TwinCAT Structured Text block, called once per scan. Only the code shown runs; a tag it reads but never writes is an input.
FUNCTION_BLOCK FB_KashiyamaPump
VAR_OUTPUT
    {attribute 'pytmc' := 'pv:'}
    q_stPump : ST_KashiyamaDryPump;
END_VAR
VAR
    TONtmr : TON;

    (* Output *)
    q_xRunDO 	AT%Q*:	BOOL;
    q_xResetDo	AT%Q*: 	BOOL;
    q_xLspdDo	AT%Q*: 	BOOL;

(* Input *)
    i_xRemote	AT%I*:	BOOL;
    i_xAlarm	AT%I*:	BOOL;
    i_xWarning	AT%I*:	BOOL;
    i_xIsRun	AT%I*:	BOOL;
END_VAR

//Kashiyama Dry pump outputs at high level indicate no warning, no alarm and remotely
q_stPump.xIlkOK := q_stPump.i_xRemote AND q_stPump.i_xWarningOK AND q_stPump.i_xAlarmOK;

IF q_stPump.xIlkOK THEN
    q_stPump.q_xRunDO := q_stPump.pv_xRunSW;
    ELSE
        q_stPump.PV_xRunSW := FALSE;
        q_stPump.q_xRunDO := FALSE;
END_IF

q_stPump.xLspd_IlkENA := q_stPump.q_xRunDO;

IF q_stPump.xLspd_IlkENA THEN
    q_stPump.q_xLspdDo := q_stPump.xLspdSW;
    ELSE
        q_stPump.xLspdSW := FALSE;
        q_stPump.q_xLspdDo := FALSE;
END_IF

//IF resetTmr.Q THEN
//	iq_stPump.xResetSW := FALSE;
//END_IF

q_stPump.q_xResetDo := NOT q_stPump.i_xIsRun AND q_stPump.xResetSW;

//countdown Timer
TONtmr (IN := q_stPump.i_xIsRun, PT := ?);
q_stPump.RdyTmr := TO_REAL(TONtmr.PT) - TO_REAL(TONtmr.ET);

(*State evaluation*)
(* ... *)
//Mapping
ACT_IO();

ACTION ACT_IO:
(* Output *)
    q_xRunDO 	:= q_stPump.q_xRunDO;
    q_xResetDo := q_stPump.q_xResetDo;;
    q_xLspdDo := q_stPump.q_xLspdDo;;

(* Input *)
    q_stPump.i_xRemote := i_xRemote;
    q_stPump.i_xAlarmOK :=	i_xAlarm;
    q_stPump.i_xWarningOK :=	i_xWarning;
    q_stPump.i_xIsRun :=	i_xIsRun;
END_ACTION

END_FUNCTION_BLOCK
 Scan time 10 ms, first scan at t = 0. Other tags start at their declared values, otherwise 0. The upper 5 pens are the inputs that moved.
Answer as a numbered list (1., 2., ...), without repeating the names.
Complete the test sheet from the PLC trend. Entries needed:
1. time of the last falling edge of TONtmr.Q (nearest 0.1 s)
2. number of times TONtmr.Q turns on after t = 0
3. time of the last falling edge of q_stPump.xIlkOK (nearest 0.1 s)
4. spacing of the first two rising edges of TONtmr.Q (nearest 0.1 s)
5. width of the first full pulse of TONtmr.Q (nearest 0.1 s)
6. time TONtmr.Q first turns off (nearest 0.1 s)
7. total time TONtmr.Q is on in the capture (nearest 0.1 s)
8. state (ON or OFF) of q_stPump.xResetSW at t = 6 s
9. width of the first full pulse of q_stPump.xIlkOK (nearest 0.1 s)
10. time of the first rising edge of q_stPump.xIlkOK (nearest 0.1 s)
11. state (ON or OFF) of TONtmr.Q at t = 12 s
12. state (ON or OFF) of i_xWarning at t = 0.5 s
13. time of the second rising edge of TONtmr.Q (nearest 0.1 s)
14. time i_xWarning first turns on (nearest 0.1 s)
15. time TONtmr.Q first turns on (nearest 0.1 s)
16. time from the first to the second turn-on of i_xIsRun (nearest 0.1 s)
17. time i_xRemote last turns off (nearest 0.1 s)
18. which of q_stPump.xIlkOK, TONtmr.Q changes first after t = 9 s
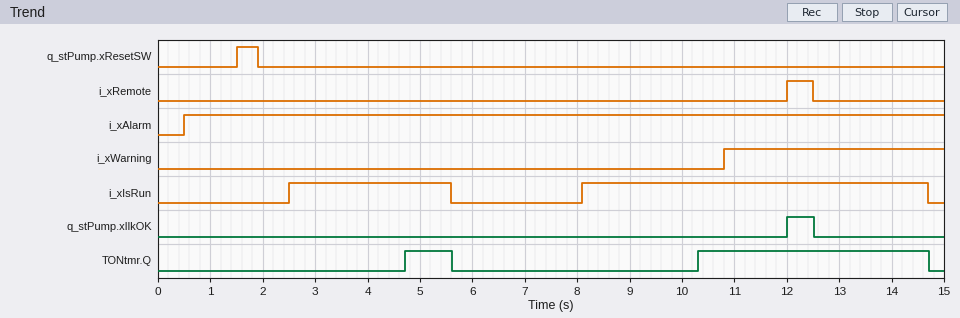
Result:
1. 14.7 s
2. 2
3. 12.5 s
4. 5.6 s
5. 0.9 s
6. 5.6 s
7. 5.3 s
8. OFF
9. 0.5 s
10. 12.0 s
11. ON
12. OFF
13. 10.3 s
14. 10.8 s
15. 4.7 s
16. 5.6 s
17. 12.5 s
18. TONtmr.Q
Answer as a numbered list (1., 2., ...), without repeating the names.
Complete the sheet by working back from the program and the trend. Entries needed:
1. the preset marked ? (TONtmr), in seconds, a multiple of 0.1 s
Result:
1. 2.2 s
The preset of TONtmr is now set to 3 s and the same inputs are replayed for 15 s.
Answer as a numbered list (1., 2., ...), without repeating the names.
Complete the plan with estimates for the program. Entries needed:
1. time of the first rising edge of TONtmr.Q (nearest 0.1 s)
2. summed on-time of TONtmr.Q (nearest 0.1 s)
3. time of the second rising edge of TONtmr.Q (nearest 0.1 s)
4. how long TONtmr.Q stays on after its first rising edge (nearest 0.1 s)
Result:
1. 5.5 s
2. 3.7 s
3. 11.1 s
4. 0.1 s
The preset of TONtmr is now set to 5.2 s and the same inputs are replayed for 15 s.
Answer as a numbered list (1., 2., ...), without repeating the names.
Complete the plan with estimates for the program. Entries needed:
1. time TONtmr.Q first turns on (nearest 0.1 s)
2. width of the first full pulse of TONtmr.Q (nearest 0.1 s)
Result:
1. 13.3 s
2. 1.4 s
